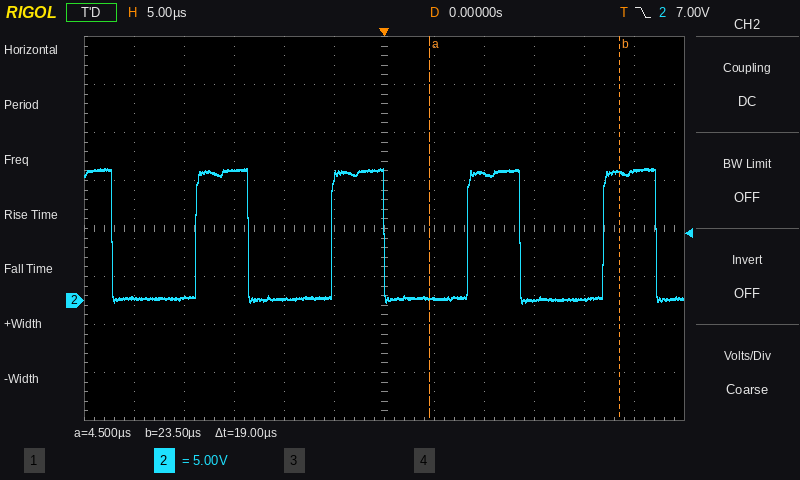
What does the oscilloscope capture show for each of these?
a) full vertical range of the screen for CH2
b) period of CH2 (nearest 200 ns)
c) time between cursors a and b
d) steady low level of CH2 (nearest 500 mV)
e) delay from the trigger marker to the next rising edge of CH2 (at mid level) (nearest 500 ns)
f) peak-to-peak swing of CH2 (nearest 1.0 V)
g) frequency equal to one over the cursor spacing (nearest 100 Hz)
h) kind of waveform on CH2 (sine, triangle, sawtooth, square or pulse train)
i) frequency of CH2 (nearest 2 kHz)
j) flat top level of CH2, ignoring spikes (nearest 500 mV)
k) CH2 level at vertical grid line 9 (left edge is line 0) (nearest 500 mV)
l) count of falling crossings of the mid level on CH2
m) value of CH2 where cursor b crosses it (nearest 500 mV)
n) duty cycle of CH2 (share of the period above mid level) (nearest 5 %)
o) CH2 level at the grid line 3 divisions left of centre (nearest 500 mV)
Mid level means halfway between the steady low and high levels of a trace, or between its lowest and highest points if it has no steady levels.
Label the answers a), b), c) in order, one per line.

a) 40 V
b) 13.6 µs
c) 19 µs
d) 0.0 V
e) 8.5 µs
f) 14.0 V
g) 52.6 kHz
h) pulse train
i) 74 kHz
j) 13.5 V
k) 0.0 V
l) 5
m) 13.5 V
n) 40 %
o) 13.5 V
